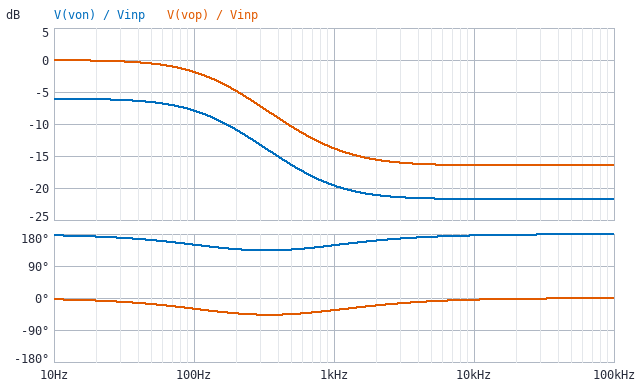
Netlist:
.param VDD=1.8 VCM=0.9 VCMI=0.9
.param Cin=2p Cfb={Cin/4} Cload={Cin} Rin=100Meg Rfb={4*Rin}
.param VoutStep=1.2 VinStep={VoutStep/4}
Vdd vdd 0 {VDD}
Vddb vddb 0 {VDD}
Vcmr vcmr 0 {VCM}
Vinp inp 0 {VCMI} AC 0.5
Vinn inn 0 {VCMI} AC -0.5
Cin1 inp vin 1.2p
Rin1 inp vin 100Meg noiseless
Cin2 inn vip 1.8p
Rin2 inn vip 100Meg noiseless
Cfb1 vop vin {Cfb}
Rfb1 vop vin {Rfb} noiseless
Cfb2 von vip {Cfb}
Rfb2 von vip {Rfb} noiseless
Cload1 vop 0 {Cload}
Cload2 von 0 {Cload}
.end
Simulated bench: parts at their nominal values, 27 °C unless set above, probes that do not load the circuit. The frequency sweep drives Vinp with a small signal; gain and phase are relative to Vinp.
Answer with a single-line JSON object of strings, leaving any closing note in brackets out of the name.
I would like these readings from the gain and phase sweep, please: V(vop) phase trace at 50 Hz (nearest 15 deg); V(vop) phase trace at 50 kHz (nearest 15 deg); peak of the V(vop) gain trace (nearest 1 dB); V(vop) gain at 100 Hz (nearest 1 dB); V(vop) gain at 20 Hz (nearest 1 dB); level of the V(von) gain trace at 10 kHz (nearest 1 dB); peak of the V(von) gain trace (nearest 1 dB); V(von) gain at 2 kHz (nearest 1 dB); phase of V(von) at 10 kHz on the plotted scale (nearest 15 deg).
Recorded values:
{"V(vop) phase trace at 50 Hz": "-15 deg", "V(vop) phase trace at 50 kHz": "0 deg", "peak of the V(vop) gain trace": "0 dB", "V(vop) gain at 100 Hz": "-2 dB", "V(vop) gain at 20 Hz": "0 dB", "level of the V(von) gain trace at 10 kHz": "-22 dB", "peak of the V(von) gain trace": "-6 dB", "V(von) gain at 2 kHz": "-21 dB", "phase of V(von) at 10 kHz on the plotted scale": "180 deg"}
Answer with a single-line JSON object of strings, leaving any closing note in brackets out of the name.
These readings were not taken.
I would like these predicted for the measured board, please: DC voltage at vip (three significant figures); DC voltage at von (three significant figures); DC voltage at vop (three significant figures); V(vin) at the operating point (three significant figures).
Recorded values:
{"DC voltage at vip": "900 mV", "DC voltage at von": "900 mV", "DC voltage at vop": "900 mV", "V(vin) at the operating point": "900 mV"}
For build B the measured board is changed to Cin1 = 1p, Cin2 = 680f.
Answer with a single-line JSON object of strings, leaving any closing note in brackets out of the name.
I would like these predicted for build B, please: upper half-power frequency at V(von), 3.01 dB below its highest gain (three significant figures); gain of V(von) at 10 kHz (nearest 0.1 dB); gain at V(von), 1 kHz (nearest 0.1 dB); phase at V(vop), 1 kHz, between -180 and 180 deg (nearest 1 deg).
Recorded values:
{"upper half-power frequency at V(von), 3.01 dB below its highest gain": "139 Hz", "gain of V(von) at 10 kHz": "-23.9 dB", "gain at V(von), 1 kHz": "-19.9 dB", "phase at V(vop), 1 kHz, between -180 and 180 deg": "-35 deg"}
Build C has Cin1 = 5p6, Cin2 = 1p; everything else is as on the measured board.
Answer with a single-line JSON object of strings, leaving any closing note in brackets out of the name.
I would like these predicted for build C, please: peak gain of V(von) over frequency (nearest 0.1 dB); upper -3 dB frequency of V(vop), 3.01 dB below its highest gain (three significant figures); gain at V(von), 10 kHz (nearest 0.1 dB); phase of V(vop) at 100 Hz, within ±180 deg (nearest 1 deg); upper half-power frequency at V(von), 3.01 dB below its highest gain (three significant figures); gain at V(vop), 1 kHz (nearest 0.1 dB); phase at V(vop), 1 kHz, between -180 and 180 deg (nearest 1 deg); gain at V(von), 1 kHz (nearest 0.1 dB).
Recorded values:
{"peak gain of V(von) over frequency": "-6.0 dB", "upper -3 dB frequency of V(vop), 3.01 dB below its highest gain": "133 Hz", "gain at V(von), 10 kHz": "-22.9 dB", "phase of V(vop) at 100 Hz, within ±180 deg": "-29 deg", "upper half-power frequency at V(von), 3.01 dB below its highest gain": "138 Hz", "gain at V(vop), 1 kHz": "-12.7 dB", "phase at V(vop), 1 kHz, between -180 and 180 deg": "-28 deg", "gain at V(von), 1 kHz": "-19.9 dB"}
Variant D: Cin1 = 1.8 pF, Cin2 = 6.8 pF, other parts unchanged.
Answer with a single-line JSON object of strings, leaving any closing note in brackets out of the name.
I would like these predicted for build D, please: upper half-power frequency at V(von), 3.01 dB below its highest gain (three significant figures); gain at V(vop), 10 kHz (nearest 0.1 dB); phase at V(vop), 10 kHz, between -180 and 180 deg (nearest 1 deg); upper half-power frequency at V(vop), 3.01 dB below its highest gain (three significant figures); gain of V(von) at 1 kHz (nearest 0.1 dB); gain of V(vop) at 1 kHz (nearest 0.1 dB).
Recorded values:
{"upper half-power frequency at V(von), 3.01 dB below its highest gain": "133 Hz", "gain at V(vop), 10 kHz": "-15.7 dB", "phase at V(vop), 10 kHz, between -180 and 180 deg": "-4 deg", "upper half-power frequency at V(vop), 3.01 dB below its highest gain": "137 Hz", "gain of V(von) at 1 kHz": "-18.6 dB", "gain of V(vop) at 1 kHz": "-13.6 dB"}
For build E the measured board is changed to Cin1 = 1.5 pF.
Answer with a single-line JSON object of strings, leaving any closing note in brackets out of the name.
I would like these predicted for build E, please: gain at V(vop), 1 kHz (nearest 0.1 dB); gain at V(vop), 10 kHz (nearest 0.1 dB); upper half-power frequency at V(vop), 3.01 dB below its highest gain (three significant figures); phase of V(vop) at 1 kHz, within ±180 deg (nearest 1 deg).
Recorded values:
{"gain at V(vop), 1 kHz": "-13.7 dB", "gain at V(vop), 10 kHz": "-16.0 dB", "upper half-power frequency at V(vop), 3.01 dB below its highest gain": "137 Hz", "phase of V(vop) at 1 kHz, within ±180 deg": "-33 deg"}
